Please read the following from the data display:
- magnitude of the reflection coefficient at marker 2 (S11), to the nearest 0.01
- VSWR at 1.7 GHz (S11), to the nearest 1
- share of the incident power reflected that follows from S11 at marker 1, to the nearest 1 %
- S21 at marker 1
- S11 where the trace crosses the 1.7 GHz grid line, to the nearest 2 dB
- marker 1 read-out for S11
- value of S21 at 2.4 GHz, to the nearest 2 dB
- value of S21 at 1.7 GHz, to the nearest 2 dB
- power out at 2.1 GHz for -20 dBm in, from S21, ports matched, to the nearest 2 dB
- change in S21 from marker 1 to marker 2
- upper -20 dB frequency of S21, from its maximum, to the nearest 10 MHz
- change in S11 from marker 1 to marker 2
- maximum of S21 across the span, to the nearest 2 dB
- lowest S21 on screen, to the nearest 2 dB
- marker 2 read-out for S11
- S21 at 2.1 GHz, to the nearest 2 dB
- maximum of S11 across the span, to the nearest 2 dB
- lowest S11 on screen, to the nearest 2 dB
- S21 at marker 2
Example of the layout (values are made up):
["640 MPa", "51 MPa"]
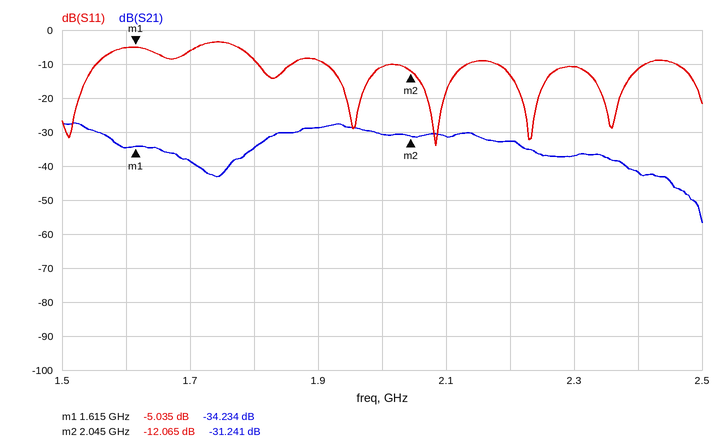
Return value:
["0.25", "3", "31 %", "-34.234 dB", "-6 dB", "-5.035 dB", "-42 dB", "-38 dB", "-52 dBm", "2.993 dB", "2.47 GHz", "-7.030 dB", "-28 dB", "-56 dB", "-12.065 dB", "-32 dB", "-4 dB", "-34 dB", "-31.241 dB"]
